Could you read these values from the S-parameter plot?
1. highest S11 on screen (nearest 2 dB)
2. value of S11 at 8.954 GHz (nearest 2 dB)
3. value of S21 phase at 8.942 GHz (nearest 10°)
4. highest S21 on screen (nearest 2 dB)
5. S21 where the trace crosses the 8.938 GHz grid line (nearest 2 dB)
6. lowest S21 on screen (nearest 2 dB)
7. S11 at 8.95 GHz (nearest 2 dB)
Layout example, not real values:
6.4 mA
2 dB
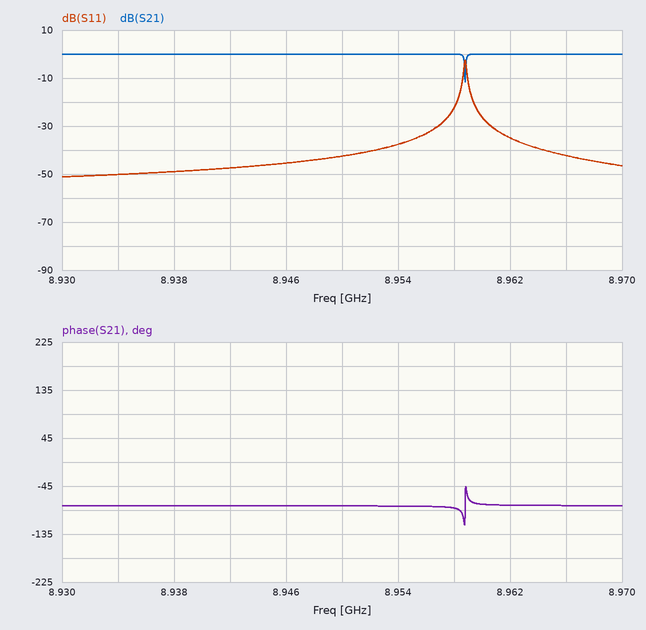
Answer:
-2 dB
-38 dB
-80°
0 dB
0 dB
-12 dB
-42 dB
